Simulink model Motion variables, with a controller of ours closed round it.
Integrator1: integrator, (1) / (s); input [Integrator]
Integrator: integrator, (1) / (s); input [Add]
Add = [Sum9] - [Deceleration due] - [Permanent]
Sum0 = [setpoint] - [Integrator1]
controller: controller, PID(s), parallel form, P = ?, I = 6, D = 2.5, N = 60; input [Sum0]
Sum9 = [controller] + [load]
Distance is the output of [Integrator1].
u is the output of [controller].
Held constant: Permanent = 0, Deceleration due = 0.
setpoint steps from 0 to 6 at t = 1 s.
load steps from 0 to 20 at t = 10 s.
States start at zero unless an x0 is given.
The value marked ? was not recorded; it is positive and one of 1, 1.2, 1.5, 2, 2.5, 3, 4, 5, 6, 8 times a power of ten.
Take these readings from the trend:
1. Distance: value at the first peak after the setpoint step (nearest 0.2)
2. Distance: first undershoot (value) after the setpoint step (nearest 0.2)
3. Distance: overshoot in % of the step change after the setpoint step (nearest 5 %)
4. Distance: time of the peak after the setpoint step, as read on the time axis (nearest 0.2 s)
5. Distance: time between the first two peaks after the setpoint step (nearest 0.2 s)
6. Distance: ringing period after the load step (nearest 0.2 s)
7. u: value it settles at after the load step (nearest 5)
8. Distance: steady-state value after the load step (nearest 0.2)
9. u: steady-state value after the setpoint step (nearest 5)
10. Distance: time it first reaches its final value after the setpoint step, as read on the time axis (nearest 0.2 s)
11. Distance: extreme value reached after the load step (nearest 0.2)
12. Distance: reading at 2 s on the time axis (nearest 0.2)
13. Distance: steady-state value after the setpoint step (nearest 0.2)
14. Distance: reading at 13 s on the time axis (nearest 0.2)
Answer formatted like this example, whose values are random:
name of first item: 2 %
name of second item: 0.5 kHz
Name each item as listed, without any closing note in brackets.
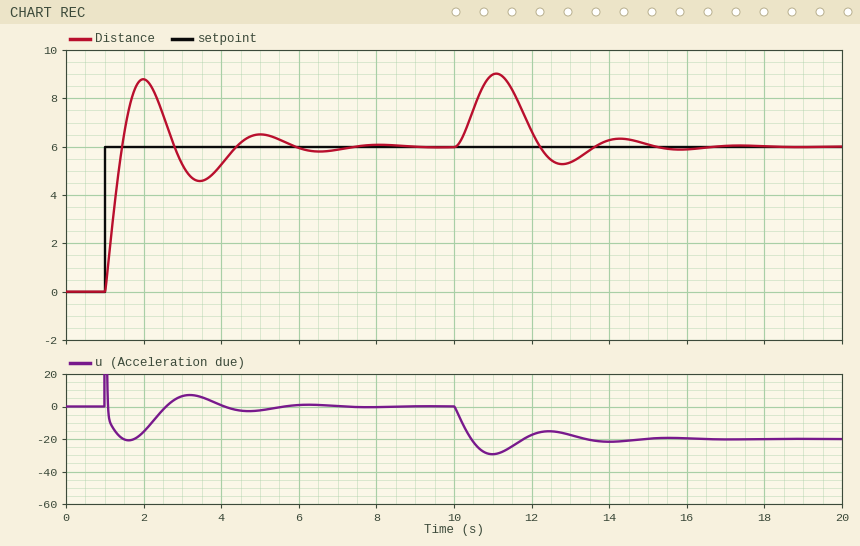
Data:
Distance: value at the first peak after the setpoint step: 8.8
Distance: first undershoot (value) after the setpoint step: 4.6
Distance: overshoot in % of the step change after the setpoint step: 45 %
Distance: time of the peak after the setpoint step, as read on the time axis: 2.0 s
Distance: time between the first two peaks after the setpoint step: 3.0 s
Distance: ringing period after the load step: 3.2 s
u: value it settles at after the load step: -20
Distance: steady-state value after the load step: 6.0
u: steady-state value after the setpoint step: 0
Distance: time it first reaches its final value after the setpoint step, as read on the time axis: 1.4 s
Distance: extreme value reached after the load step: 9.0
Distance: reading at 2 s on the time axis: 8.8
Distance: steady-state value after the setpoint step: 6.0
Distance: reading at 13 s on the time axis: 5.4
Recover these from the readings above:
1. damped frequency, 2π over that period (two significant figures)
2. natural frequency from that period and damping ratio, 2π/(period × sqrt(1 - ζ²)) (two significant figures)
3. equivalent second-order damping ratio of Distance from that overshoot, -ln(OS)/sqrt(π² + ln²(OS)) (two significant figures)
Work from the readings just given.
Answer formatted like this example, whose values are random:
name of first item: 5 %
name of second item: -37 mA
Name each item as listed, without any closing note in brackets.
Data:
damped frequency, 2π over that period: 2.1 rad/s
natural frequency from that period and damping ratio, 2π/(period × sqrt(1 - ζ²)): 2.2 rad/s
equivalent second-order damping ratio of Distance from that overshoot, -ln(OS)/sqrt(π² + ln²(OS)): 0.25
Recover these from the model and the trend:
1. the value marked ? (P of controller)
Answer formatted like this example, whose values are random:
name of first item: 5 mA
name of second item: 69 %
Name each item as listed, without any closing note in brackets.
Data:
the value marked ?: 6
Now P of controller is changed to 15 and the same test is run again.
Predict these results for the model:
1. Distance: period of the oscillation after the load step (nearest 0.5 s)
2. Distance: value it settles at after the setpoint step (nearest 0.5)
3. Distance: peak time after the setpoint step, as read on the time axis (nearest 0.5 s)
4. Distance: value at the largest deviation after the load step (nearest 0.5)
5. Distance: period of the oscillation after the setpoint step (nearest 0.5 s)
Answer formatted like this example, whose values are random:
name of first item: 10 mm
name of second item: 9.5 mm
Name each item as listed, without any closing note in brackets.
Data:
Distance: period of the oscillation after the load step: 1.5 s
Distance: value it settles at after the setpoint step: 6.0
Distance: peak time after the setpoint step, as read on the time axis: 1.5 s
Distance: value at the largest deviation after the load step: 7.5
Distance: period of the oscillation after the setpoint step: 1.5 s
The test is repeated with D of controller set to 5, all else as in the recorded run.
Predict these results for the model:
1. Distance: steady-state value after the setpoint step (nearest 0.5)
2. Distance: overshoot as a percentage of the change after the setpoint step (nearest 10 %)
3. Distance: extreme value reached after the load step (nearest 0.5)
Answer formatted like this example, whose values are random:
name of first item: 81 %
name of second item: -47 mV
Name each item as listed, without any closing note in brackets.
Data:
Distance: steady-state value after the setpoint step: 6.0
Distance: overshoot as a percentage of the change after the setpoint step: 20 %
Distance: extreme value reached after the load step: 8.0
